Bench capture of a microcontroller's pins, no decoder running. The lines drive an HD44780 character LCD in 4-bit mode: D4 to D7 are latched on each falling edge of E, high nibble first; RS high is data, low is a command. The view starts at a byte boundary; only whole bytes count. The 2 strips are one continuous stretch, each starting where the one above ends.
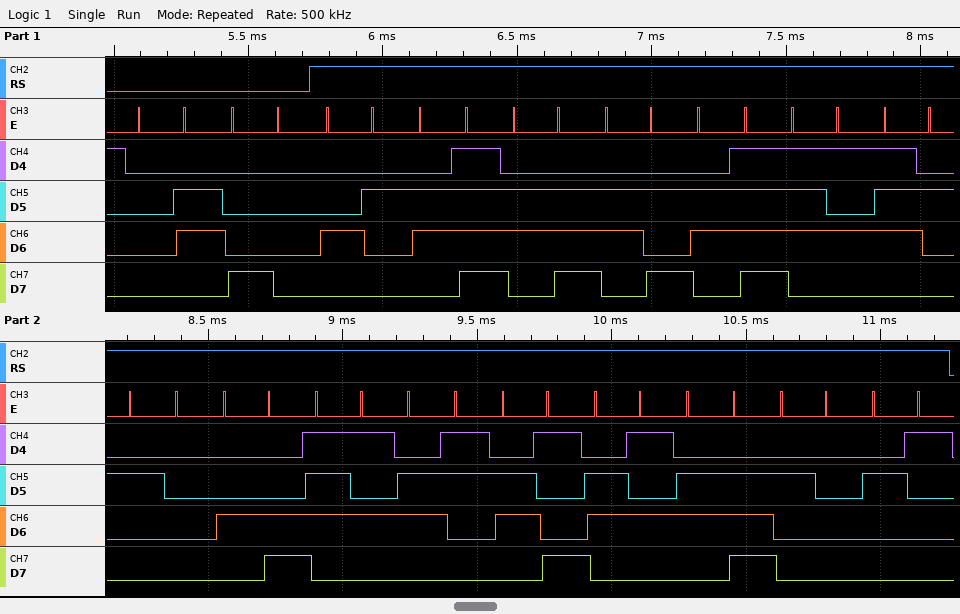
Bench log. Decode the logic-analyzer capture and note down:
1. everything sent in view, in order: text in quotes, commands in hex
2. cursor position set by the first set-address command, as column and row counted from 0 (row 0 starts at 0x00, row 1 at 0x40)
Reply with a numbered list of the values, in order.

1. 0x06 0x80 "Bonjour Lucien !"
2. column 0, row 0
